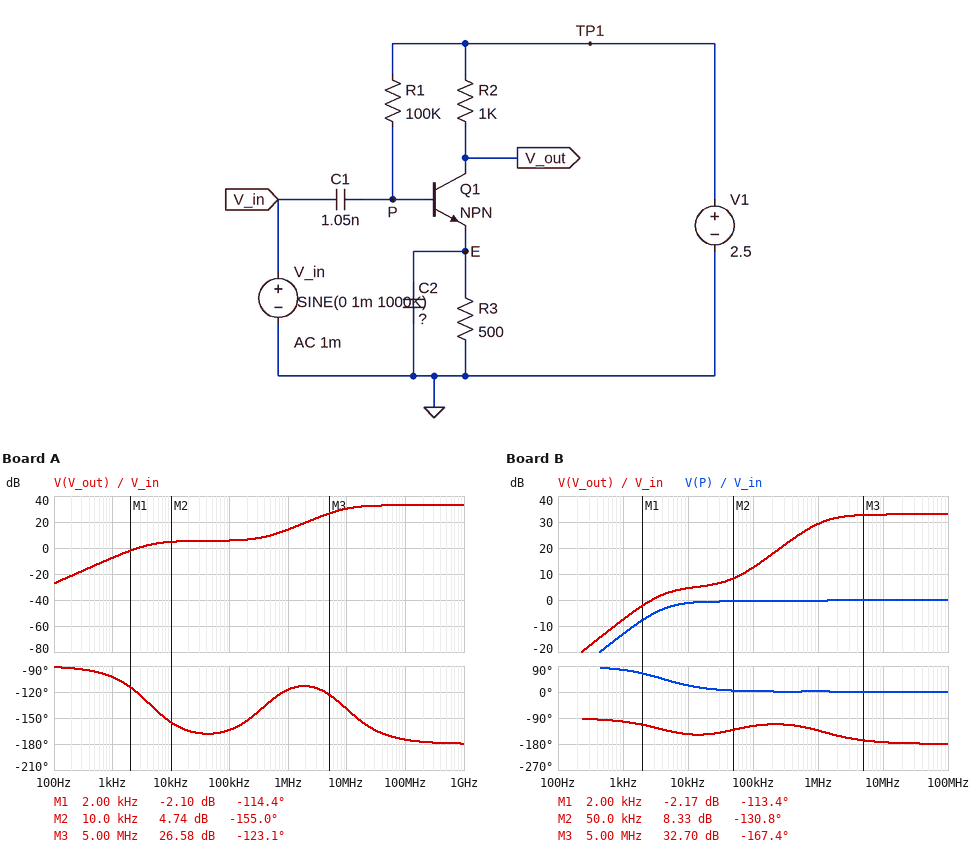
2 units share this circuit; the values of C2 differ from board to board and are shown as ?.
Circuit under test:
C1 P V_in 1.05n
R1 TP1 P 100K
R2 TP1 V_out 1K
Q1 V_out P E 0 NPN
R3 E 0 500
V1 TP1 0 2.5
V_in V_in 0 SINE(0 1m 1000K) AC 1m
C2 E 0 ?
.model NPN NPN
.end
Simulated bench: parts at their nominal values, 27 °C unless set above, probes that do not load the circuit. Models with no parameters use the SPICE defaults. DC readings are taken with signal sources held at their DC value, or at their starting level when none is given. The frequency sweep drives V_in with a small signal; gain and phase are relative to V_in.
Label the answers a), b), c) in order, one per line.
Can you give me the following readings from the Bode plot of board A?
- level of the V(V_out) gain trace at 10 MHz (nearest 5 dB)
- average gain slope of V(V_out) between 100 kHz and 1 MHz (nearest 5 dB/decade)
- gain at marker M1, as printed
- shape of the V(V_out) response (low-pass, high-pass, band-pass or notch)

a) 30 dB
b) 10 dB/decade
c) -2.10 dB
d) high-pass
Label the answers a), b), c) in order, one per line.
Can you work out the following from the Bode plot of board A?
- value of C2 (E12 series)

a) 820 pF
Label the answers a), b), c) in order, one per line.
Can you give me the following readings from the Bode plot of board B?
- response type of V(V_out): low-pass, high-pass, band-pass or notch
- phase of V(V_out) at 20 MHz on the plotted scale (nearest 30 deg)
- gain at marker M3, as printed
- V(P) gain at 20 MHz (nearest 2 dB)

a) high-pass
b) -180 deg
c) 32.70 dB
d) 0 dB
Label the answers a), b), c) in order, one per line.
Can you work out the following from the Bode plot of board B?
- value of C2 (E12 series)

a) 6.8 nF
